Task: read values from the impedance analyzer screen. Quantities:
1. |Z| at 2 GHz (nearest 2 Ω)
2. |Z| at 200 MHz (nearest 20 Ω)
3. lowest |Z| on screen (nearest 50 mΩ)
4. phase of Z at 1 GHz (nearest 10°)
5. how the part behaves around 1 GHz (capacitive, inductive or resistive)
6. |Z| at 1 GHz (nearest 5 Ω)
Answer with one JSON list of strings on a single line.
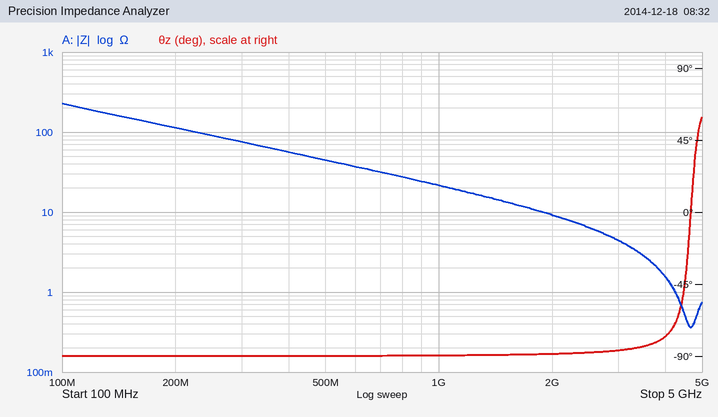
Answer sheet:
["10 Ω", "120 Ω", "350 mΩ", "-90°", "capacitive", "20 Ω"]
